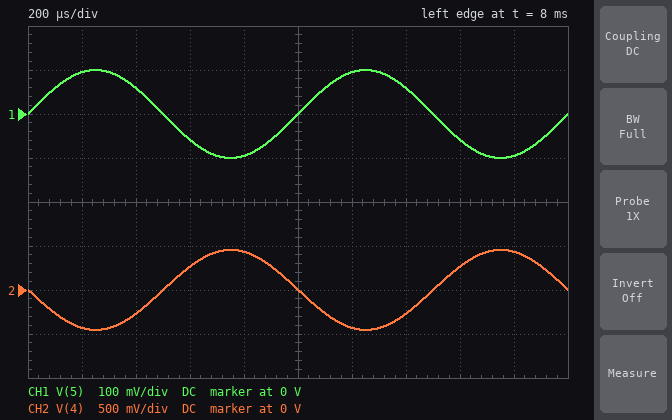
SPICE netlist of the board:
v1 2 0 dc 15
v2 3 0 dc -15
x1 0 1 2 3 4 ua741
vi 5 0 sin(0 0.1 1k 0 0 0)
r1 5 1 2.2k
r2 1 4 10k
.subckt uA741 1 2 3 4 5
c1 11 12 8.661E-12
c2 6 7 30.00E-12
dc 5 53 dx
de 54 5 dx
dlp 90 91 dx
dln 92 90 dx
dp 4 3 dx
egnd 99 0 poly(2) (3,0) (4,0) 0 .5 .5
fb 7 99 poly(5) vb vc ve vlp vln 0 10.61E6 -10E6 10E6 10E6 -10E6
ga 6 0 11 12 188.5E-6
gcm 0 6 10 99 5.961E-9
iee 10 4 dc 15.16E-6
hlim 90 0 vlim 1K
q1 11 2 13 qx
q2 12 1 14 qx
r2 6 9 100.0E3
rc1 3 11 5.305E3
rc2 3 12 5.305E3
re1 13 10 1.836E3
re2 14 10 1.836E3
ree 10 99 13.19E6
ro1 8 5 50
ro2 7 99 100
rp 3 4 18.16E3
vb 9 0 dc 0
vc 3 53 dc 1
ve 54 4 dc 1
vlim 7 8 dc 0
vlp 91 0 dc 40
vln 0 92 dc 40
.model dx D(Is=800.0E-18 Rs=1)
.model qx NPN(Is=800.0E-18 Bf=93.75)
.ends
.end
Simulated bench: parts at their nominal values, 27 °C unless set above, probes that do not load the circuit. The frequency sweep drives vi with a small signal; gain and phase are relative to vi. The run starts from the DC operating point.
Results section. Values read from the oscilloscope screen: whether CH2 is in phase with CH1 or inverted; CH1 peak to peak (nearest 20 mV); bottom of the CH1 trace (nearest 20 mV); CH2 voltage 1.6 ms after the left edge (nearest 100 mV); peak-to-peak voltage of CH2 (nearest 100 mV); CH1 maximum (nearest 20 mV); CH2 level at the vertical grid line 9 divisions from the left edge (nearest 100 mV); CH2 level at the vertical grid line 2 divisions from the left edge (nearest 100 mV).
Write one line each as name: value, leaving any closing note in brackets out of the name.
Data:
whether CH2 is in phase with CH1 or inverted: inverted
CH1 peak to peak: 200 mV
bottom of the CH1 trace: -100 mV
CH2 voltage 1.6 ms after the left edge: 300 mV
peak-to-peak voltage of CH2: 900 mV
CH1 maximum: 100 mV
CH2 level at the vertical grid line 9 divisions from the left edge: 400 mV
CH2 level at the vertical grid line 2 divisions from the left edge: -300 mV
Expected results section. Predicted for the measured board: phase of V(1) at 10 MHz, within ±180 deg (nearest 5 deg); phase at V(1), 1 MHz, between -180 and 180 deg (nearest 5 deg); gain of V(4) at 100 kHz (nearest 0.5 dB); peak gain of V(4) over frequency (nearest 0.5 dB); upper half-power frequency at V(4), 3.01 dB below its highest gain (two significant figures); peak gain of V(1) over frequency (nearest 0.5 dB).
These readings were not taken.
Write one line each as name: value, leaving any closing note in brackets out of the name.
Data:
phase of V(1) at 10 MHz, within ±180 deg: 0 deg
phase at V(1), 1 MHz, between -180 and 180 deg: 10 deg
gain of V(4) at 100 kHz: 12.0 dB
peak gain of V(4) over frequency: 13.0 dB
upper half-power frequency at V(4), 3.01 dB below its highest gain: 200 kHz
peak gain of V(1) over frequency: -1.0 dB
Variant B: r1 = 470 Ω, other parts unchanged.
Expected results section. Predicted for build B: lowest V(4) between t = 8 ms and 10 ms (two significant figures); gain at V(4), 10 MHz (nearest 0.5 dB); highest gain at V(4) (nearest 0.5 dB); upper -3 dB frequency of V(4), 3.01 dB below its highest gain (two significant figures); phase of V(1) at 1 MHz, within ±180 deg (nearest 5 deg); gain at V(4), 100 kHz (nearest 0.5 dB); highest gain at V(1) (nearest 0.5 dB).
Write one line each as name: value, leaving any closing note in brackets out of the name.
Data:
lowest V(4) between t = 8 ms and 10 ms: -2.1 V
gain at V(4), 10 MHz: -33.5 dB
highest gain at V(4): 26.5 dB
upper -3 dB frequency of V(4), 3.01 dB below its highest gain: 46 kHz
phase of V(1) at 1 MHz, within ±180 deg: 0 deg
gain at V(4), 100 kHz: 19.0 dB
highest gain at V(1): 0 dB
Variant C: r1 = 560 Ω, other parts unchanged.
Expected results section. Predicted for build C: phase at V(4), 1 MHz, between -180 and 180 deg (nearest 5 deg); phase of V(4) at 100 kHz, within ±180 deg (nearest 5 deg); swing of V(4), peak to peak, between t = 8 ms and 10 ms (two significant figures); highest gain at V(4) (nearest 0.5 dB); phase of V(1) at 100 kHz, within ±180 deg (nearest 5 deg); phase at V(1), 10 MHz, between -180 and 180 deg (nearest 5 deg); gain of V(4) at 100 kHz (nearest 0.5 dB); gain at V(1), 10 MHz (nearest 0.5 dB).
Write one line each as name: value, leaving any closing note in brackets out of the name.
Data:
phase at V(4), 1 MHz, between -180 and 180 deg: 60 deg
phase of V(4) at 100 kHz, within ±180 deg: 115 deg
swing of V(4), peak to peak, between t = 8 ms and 10 ms: 3.6 V
highest gain at V(4): 25.0 dB
phase of V(1) at 100 kHz, within ±180 deg: 30 deg
phase at V(1), 10 MHz, between -180 and 180 deg: 0 deg
gain of V(4) at 100 kHz: 18.5 dB
gain at V(1), 10 MHz: -0.5 dB
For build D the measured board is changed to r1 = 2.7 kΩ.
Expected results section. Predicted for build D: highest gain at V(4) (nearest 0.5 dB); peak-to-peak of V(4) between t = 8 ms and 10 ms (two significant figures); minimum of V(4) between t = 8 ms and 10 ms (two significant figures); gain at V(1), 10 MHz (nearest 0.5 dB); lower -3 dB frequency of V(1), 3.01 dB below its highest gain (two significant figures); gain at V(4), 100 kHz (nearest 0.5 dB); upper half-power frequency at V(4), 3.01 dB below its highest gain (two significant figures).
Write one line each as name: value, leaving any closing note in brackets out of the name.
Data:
highest gain at V(4): 11.5 dB
peak-to-peak of V(4) between t = 8 ms and 10 ms: 740 mV
minimum of V(4) between t = 8 ms and 10 ms: -370 mV
gain at V(1), 10 MHz: -2.0 dB
lower -3 dB frequency of V(1), 3.01 dB below its highest gain: 220 kHz
gain at V(4), 100 kHz: 10.5 dB
upper half-power frequency at V(4), 3.01 dB below its highest gain: 240 kHz
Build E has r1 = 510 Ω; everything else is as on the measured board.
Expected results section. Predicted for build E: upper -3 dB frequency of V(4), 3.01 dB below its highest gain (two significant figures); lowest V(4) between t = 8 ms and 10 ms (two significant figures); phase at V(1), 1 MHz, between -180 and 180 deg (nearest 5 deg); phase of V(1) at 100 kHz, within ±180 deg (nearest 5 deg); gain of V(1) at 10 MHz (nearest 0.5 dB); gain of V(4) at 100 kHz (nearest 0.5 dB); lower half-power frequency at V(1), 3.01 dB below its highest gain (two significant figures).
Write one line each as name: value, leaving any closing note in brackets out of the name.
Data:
upper -3 dB frequency of V(4), 3.01 dB below its highest gain: 50 kHz
lowest V(4) between t = 8 ms and 10 ms: -2.0 V
phase at V(1), 1 MHz, between -180 and 180 deg: 0 deg
phase of V(1) at 100 kHz, within ±180 deg: 25 deg
gain of V(1) at 10 MHz: -0.5 dB
gain of V(4) at 100 kHz: 19.0 dB
lower half-power frequency at V(1), 3.01 dB below its highest gain: 49 kHz
